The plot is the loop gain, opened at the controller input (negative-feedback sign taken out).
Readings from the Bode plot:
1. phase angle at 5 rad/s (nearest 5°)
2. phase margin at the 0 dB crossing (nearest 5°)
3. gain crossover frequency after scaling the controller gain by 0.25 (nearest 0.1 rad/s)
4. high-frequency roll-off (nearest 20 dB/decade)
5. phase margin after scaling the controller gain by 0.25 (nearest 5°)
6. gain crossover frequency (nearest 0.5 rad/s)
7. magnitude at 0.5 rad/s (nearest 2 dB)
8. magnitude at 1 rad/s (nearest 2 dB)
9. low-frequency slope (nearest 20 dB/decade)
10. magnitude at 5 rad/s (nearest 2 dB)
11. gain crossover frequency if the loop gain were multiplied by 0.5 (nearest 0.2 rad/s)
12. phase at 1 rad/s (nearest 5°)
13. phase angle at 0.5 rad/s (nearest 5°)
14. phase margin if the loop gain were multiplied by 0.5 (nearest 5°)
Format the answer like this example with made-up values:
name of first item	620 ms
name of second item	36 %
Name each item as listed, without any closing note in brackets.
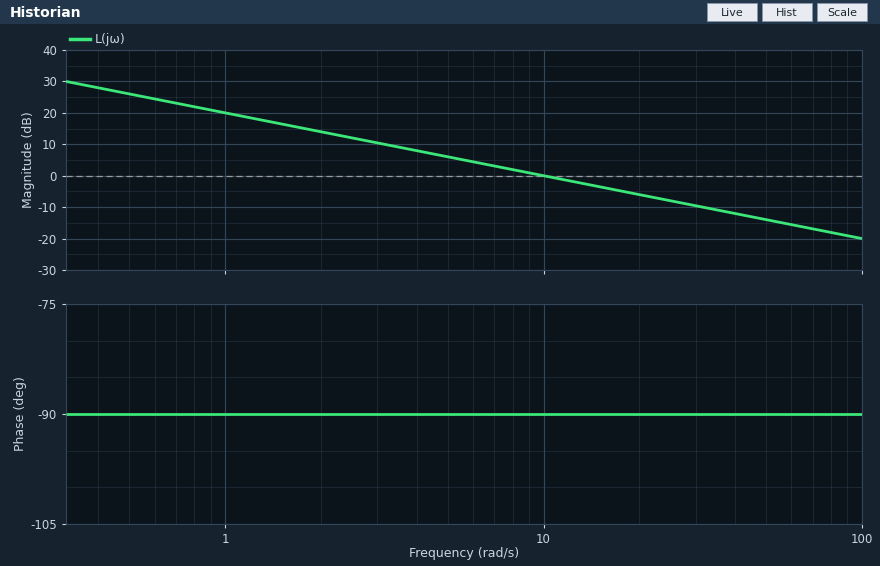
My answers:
phase angle at 5 rad/s	-90°
phase margin at the 0 dB crossing	90°
gain crossover frequency after scaling the controller gain by 0.25	2.5 rad/s
high-frequency roll-off	-20 dB/decade
phase margin after scaling the controller gain by 0.25	90°
gain crossover frequency	10.0 rad/s
magnitude at 0.5 rad/s	26 dB
magnitude at 1 rad/s	20 dB
low-frequency slope	-20 dB/decade
magnitude at 5 rad/s	6 dB
gain crossover frequency if the loop gain were multiplied by 0.5	5.0 rad/s
phase at 1 rad/s	-90°
phase angle at 0.5 rad/s	-90°
phase margin if the loop gain were multiplied by 0.5	90°
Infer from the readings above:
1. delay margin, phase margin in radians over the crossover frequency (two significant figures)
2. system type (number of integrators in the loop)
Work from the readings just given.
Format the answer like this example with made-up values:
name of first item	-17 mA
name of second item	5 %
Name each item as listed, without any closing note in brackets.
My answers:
delay margin, phase margin in radians over the crossover frequency	0.16 s
system type	1
